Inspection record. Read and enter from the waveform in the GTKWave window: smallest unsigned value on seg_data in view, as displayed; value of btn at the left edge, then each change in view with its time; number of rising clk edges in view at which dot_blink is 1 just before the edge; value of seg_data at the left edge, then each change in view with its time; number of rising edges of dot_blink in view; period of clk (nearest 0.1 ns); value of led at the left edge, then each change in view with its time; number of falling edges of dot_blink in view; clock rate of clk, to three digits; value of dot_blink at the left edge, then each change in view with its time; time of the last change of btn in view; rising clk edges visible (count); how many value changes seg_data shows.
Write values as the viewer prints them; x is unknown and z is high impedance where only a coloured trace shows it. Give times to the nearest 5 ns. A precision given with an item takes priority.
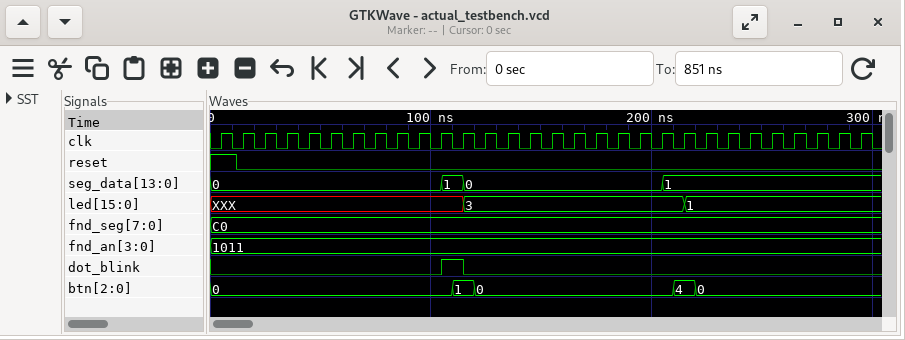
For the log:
0
0, 1 at 110 ns, 0 at 120 ns, 4 at 210 ns, 0 at 220 ns
1
0, 1 at 105 ns, 0 at 115 ns, 1 at 205 ns
1
10 ns
XXX, 3 at 115 ns, 1 at 215 ns
1
100 MHz
0, 1 at 105 ns, 0 at 115 ns
220 ns
30
3
